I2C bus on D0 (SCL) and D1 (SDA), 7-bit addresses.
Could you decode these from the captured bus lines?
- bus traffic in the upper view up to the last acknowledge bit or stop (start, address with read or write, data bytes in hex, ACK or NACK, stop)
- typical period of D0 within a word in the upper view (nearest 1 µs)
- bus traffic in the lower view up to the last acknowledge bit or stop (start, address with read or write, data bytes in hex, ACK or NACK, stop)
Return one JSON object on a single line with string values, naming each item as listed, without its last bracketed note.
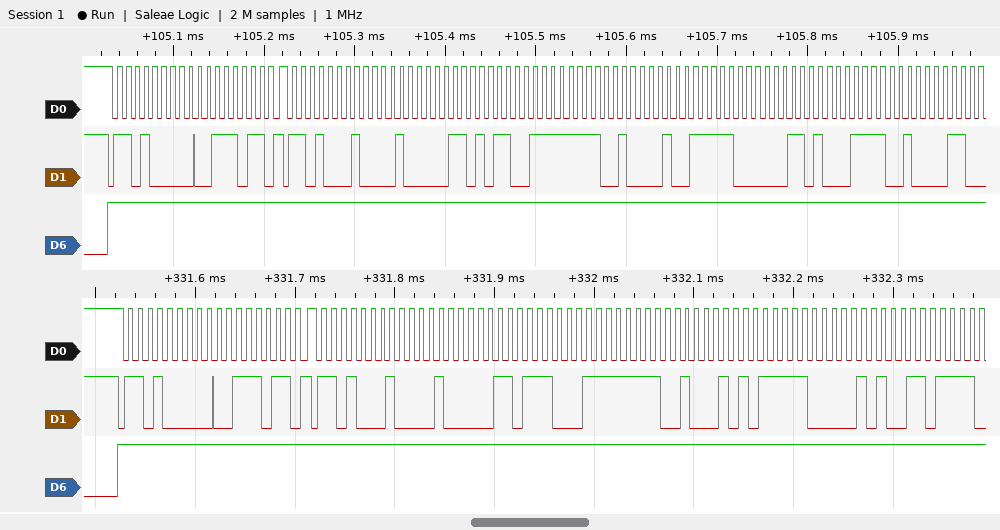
{"bus traffic in the upper view up to the last acknowledge bit or stop": "start, address 68 write ACK, 3B ACK, repeated start, address 68 read ACK, 10 ACK, D6 ACK, FF ACK, 42 ACK, F8 ACK, 34 ACK, F2 ACK", "typical period of D0 within a word in the upper view": "10 µs", "bus traffic in the lower view up to the last acknowledge bit or stop": "start, address 68 write ACK, 3B ACK, repeated start, address 68 read ACK, 10 ACK, DC ACK, FF ACK, 45 ACK, F8 ACK, 53 ACK"}
